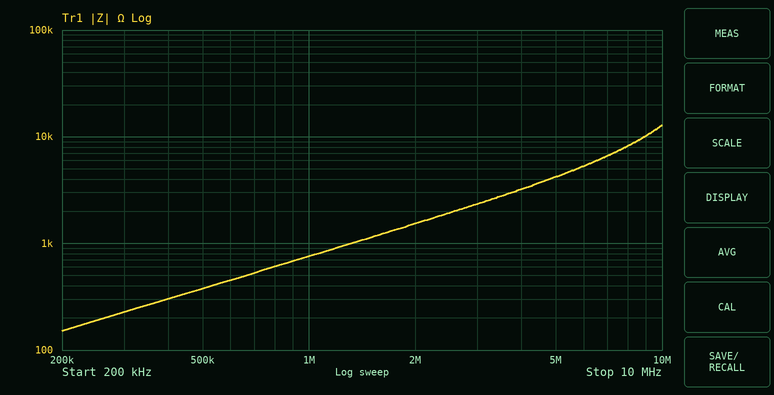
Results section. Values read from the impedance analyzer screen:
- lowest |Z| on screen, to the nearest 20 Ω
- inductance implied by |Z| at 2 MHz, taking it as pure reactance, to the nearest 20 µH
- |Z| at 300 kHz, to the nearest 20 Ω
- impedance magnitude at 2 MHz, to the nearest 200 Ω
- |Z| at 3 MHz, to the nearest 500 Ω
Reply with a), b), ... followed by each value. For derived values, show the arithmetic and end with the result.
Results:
a) 160 Ω
b) L = 1.6 kΩ/(2π × 2 MHz) ≈ 127 µH, so 120 µH to the nearest 20 µH
c) 220 Ω
d) 1.6 kΩ
e) 2.5 kΩ
